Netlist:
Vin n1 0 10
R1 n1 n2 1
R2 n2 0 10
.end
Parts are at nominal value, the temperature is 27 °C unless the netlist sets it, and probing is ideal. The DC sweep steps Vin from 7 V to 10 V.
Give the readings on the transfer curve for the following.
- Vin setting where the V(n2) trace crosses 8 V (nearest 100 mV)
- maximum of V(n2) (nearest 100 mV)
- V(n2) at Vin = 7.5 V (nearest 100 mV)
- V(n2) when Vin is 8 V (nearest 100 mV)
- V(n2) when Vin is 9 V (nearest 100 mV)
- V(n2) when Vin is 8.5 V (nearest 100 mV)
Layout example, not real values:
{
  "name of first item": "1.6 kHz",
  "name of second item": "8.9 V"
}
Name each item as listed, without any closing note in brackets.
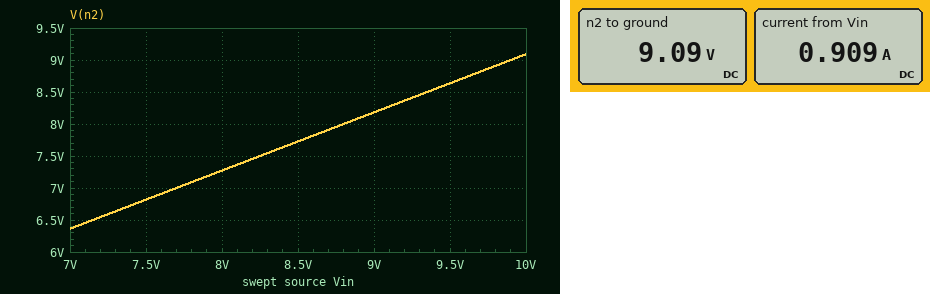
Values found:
{
  "Vin setting where the V(n2) trace crosses 8 V": "8.8 V",
  "maximum of V(n2)": "9.1 V",
  "V(n2) at Vin = 7.5 V": "6.8 V",
  "V(n2) when Vin is 8 V": "7.3 V",
  "V(n2) when Vin is 9 V": "8.2 V",
  "V(n2) when Vin is 8.5 V": "7.7 V"
}
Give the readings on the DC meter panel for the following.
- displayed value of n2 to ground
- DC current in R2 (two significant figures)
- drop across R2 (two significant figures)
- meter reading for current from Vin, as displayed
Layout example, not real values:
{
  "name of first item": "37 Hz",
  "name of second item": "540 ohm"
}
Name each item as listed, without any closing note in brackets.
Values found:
{
  "displayed value of n2 to ground": "9.09 V",
  "DC current in R2": "910 mA",
  "drop across R2": "9.1 V",
  "meter reading for current from Vin, as displayed": "0.909 A"
}
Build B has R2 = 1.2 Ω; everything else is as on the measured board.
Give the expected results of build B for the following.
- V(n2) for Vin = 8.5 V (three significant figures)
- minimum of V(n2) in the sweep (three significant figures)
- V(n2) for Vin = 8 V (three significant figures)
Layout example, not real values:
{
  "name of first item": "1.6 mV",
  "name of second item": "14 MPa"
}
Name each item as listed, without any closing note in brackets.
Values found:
{
  "V(n2) for Vin = 8.5 V": "4.64 V",
  "minimum of V(n2) in the sweep": "3.82 V",
  "V(n2) for Vin = 8 V": "4.36 V"
}
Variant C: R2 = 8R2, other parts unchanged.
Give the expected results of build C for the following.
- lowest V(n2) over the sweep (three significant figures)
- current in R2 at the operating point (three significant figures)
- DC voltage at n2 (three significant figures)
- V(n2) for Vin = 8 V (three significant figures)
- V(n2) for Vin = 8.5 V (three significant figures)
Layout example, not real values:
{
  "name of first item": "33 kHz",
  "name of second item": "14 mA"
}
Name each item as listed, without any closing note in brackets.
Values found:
{
  "lowest V(n2) over the sweep": "6.24 V",
  "current in R2 at the operating point": "1.09 A",
  "DC voltage at n2": "8.91 V",
  "V(n2) for Vin = 8 V": "7.13 V",
  "V(n2) for Vin = 8.5 V": "7.58 V"
}
